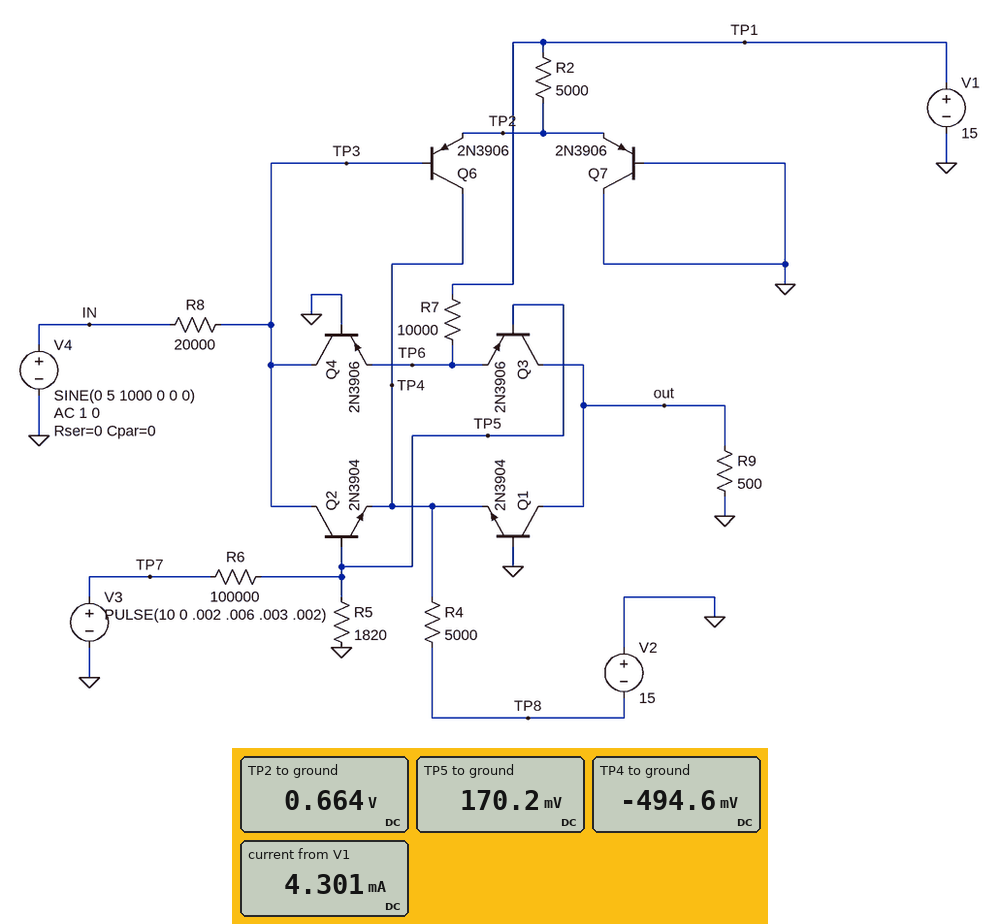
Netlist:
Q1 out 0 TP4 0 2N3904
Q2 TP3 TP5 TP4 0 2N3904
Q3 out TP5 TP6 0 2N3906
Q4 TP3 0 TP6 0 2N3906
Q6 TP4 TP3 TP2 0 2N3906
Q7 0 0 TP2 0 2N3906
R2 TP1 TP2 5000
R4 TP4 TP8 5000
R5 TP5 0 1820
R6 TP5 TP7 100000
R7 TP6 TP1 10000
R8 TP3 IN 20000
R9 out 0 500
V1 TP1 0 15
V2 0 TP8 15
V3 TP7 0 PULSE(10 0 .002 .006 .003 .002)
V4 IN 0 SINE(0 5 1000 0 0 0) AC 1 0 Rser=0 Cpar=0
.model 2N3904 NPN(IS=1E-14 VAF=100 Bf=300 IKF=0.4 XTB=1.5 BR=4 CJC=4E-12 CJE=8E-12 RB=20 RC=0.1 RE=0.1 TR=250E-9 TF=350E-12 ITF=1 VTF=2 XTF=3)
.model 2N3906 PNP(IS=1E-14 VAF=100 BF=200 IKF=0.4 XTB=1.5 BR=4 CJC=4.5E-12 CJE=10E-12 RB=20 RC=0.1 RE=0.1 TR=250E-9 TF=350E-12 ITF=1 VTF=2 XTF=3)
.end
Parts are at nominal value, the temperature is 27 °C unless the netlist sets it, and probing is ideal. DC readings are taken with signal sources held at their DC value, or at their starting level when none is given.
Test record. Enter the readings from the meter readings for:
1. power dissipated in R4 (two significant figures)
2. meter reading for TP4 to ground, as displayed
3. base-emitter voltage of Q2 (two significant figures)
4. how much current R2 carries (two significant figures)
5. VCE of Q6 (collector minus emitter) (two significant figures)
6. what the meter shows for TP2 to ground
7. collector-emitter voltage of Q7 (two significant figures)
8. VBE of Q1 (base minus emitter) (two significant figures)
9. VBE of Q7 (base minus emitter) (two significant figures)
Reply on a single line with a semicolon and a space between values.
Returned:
42 mW; -494.6 mV; 660 mV; 2.9 mA; -1.2 V; 0.664 V; -660 mV; 490 mV; -660 mV
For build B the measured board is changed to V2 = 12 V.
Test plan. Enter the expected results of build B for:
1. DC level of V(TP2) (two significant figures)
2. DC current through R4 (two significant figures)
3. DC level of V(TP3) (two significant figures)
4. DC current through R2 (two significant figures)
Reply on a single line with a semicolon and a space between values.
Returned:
670 mV; 2.3 mA; 22 mV; 2.9 mA
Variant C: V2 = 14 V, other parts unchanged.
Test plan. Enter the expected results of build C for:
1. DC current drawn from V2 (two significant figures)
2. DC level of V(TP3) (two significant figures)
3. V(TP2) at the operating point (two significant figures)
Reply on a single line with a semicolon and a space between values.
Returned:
2.7 mA; 6.1 mV; 670 mV
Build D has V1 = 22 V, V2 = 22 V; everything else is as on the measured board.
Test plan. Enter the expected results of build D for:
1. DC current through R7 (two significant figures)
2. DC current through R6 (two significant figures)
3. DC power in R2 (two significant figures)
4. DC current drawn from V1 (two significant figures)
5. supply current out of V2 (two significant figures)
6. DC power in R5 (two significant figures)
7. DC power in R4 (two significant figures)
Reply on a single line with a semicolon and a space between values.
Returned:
2.1 mA; 98 µA; 91 mW; 6.4 mA; 4.3 mA; 15 µW; 92 mW
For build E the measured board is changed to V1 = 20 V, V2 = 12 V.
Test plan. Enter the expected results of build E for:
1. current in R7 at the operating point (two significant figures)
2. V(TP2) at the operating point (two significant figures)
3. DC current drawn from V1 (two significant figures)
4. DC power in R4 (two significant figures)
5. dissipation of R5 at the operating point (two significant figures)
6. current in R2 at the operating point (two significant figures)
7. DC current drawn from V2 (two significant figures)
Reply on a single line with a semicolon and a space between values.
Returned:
1.9 mA; 690 mV; 5.8 mA; 26 mW; 15 µW; 3.9 mA; 2.3 mA
